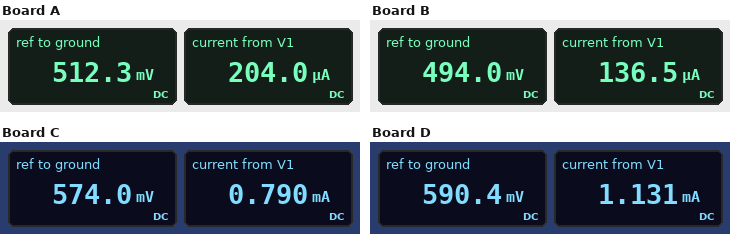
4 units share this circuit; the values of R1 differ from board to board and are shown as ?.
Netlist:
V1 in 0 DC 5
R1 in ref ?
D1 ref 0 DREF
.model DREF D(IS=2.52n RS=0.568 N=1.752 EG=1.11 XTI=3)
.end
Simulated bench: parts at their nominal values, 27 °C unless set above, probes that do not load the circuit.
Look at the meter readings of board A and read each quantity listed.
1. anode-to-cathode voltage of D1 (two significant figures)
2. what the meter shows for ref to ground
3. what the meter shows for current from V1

510 mV
512.3 mV
204.0 µA
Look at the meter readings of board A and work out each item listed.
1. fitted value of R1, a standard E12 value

22 kΩ
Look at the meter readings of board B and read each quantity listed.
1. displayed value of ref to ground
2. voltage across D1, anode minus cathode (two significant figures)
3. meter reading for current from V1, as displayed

494.0 mV
490 mV
136.5 µA
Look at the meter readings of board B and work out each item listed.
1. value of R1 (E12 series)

33 kΩ
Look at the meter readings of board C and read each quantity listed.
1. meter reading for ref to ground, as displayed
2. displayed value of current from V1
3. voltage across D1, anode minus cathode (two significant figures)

574.0 mV
0.790 mA
570 mV
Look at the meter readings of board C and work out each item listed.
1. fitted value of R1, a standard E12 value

5.6 kΩ
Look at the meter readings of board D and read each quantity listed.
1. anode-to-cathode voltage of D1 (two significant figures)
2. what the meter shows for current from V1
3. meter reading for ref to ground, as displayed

590 mV
1.131 mA
590.4 mV
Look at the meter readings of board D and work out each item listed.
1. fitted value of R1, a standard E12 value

3.9 kΩ
